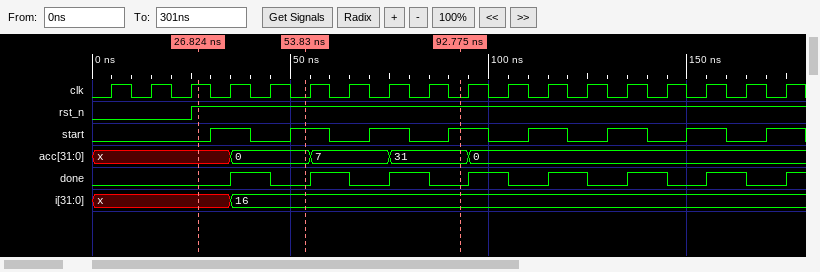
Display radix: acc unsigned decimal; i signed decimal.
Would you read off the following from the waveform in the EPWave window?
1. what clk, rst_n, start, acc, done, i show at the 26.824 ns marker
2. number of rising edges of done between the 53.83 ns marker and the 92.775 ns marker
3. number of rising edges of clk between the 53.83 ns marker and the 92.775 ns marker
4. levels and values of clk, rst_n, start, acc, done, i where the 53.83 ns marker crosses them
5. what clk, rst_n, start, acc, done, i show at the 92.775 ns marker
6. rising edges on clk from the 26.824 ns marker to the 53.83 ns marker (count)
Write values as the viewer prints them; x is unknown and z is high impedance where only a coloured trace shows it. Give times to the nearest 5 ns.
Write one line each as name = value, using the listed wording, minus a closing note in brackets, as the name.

what clk, rst_n, start, acc, done, i show at the 26.824 ns marker = clk=1, rst_n=1, start=0, acc=x, done=0, i=x
number of rising edges of done between the 53.83 ns marker and the 92.775 ns marker = 2
number of rising edges of clk between the 53.83 ns marker and the 92.775 ns marker = 4
levels and values of clk, rst_n, start, acc, done, i where the 53.83 ns marker crosses them = clk=0, rst_n=1, start=1, acc=0, done=0, i=16
what clk, rst_n, start, acc, done, i show at the 92.775 ns marker = clk=0, rst_n=1, start=1, acc=31, done=0, i=16
rising edges on clk from the 26.824 ns marker to the 53.83 ns marker = 2
